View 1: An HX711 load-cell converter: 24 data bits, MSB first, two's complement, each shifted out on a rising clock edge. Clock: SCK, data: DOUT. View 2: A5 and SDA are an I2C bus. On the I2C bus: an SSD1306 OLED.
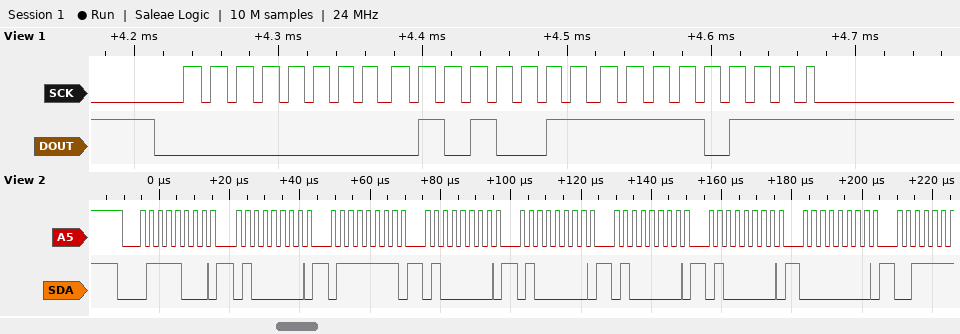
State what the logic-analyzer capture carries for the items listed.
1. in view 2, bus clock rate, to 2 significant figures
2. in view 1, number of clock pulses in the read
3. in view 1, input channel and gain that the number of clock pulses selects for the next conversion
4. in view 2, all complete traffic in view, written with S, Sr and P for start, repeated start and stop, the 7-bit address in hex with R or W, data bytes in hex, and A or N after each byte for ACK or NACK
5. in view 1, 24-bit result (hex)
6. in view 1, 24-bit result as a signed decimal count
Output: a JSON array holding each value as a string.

["400 kHz", "25", "channel A, gain 128", "S 3CW A 40 A 7F A 40 A 40 A 40 A 40 A 00 A", "0x0053F7", "21495"]
